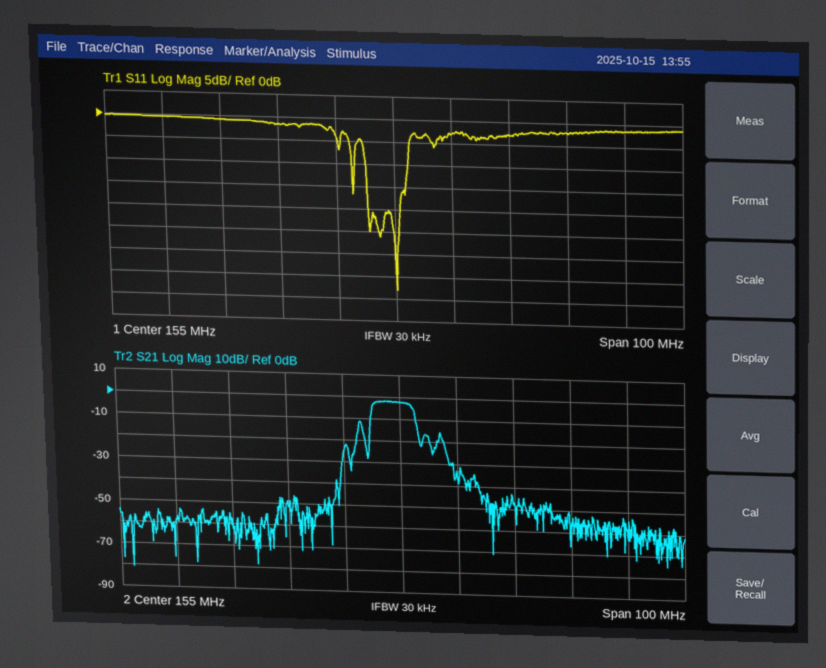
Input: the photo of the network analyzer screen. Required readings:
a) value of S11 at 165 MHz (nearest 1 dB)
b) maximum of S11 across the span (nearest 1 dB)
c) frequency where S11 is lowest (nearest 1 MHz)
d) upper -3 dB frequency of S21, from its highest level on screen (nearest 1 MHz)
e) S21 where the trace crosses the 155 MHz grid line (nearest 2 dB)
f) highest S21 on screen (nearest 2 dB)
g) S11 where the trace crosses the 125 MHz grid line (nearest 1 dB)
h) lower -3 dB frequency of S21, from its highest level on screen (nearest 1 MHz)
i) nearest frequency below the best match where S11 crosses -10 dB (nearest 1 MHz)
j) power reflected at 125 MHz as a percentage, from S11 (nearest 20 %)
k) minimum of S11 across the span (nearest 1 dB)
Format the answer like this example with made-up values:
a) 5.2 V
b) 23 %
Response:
a) -3 dB
b) 0 dB
c) 155 MHz
d) 157 MHz
e) -2 dB
f) -2 dB
g) -1 dB
h) 150 MHz
i) 150 MHz
j) 80 %
k) -38 dB
